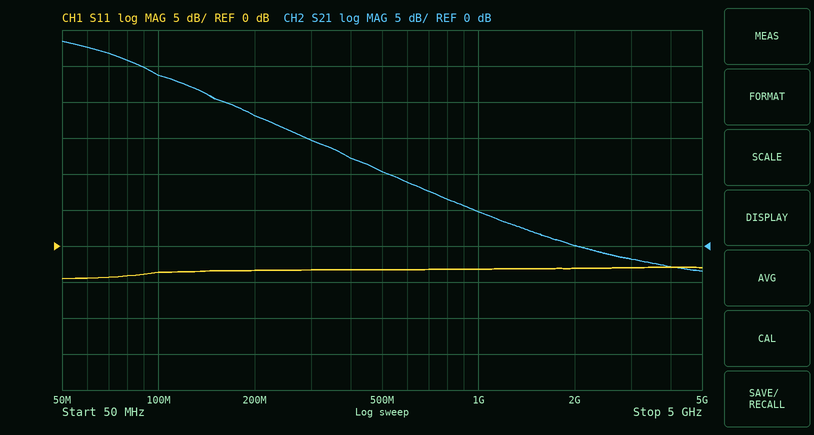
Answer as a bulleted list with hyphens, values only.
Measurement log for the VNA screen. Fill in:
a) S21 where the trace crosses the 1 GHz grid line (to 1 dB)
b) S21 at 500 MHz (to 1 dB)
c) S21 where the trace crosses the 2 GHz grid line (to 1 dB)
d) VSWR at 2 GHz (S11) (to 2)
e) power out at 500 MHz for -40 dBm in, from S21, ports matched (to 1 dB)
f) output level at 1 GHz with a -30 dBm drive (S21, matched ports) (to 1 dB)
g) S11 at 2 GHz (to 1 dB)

- 5 dB
- 10 dB
- 0 dB
- 6
- -30 dBm
- -25 dBm
- -3 dB
